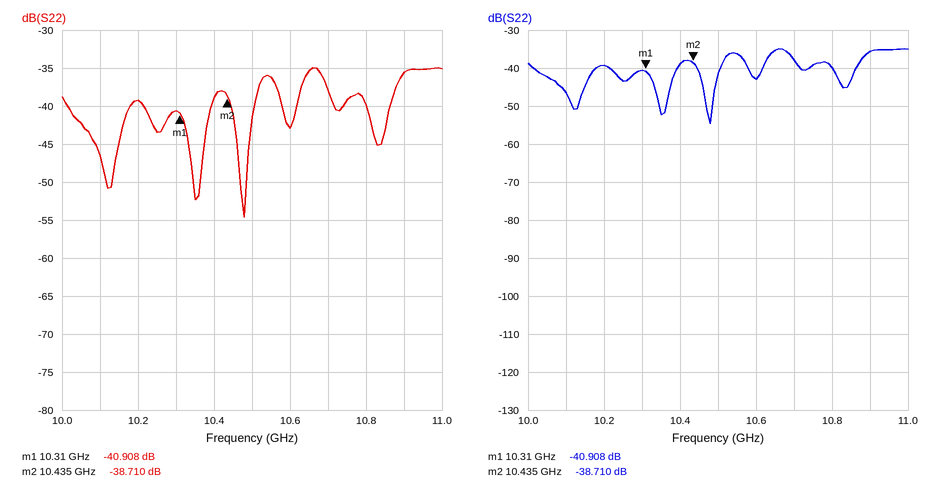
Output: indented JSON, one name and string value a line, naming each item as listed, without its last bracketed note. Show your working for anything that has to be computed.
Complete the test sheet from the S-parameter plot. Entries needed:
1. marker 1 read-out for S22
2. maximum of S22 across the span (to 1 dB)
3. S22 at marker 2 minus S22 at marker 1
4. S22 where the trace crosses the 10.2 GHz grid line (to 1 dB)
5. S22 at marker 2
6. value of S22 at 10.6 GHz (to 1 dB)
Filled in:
{
  "marker 1 read-out for S22": "-40.908 dB",
  "maximum of S22 across the span": "-35 dB",
  "S22 at marker 2 minus S22 at marker 1": "-38.71 − (-40.908) = 2.198 dB",
  "S22 where the trace crosses the 10.2 GHz grid line": "-39 dB",
  "S22 at marker 2": "-38.710 dB",
  "value of S22 at 10.6 GHz": "-43 dB"
}
